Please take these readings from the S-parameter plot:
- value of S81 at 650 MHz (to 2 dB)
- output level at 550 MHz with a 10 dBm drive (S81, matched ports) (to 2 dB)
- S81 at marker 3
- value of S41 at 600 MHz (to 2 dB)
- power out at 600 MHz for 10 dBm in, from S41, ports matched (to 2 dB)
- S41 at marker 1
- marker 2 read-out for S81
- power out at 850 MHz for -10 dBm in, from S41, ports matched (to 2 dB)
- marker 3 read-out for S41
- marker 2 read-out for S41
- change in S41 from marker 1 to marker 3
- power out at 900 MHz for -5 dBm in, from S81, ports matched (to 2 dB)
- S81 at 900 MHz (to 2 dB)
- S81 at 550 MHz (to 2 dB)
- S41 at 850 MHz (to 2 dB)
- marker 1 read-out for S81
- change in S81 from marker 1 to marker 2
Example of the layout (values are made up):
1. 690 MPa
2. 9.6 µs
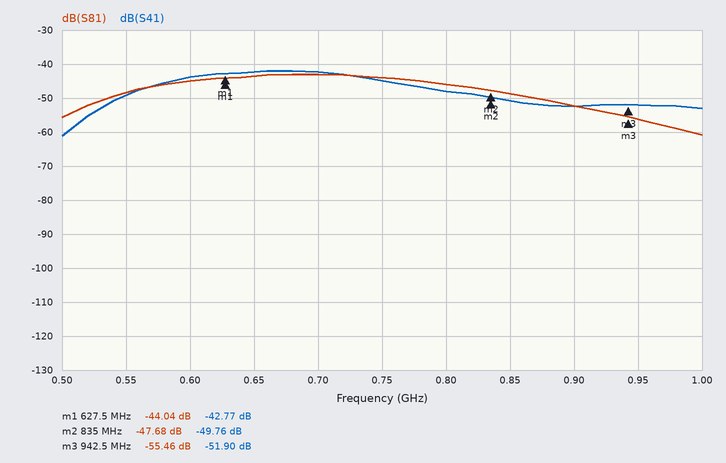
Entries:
1. -44 dB
2. -38 dBm
3. -55.46 dB
4. -44 dB
5. -34 dBm
6. -42.77 dB
7. -47.68 dB
8. -60 dBm
9. -51.90 dB
10. -49.76 dB
11. -9.13 dB
12. -58 dBm
13. -52 dB
14. -48 dB
15. -50 dB
16. -44.04 dB
17. -3.64 dB
